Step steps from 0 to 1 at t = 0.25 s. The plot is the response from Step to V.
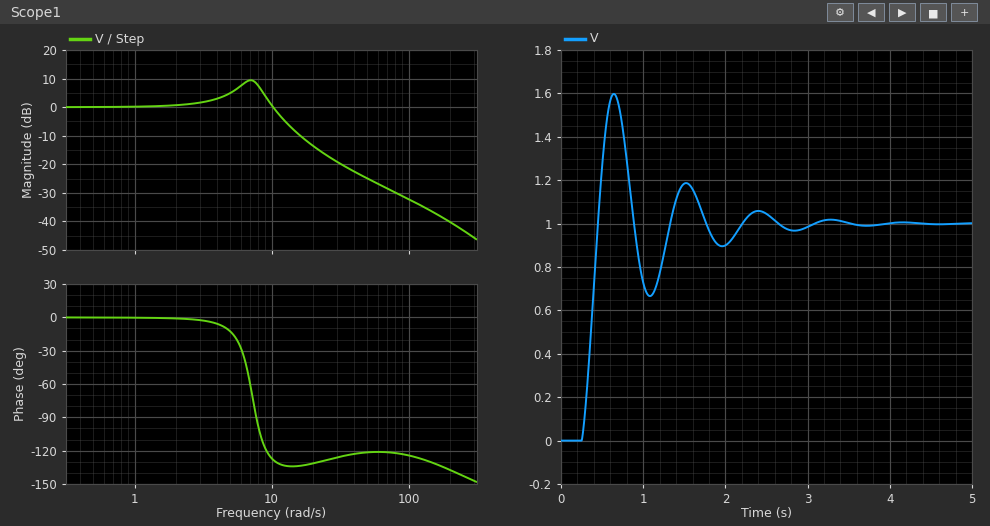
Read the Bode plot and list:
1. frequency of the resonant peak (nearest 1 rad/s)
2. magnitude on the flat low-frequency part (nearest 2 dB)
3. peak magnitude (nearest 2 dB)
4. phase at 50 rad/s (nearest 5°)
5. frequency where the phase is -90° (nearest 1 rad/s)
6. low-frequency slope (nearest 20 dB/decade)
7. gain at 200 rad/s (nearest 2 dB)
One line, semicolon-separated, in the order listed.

7 rad/s; 0 dB; 10 dB; -120°; 8 rad/s; 0 dB/decade; -40 dB
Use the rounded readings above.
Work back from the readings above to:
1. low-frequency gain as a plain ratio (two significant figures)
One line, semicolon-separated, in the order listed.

1.0
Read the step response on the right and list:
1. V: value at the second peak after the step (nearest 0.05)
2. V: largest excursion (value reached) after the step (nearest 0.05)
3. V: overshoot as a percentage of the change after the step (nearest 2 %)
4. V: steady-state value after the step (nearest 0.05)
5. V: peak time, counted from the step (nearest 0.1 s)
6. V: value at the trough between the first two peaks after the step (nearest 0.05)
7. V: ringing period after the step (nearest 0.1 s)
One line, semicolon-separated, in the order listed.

1.20; 1.60; 60 %; 1.00; 0.4 s; 0.65; 0.9 s
